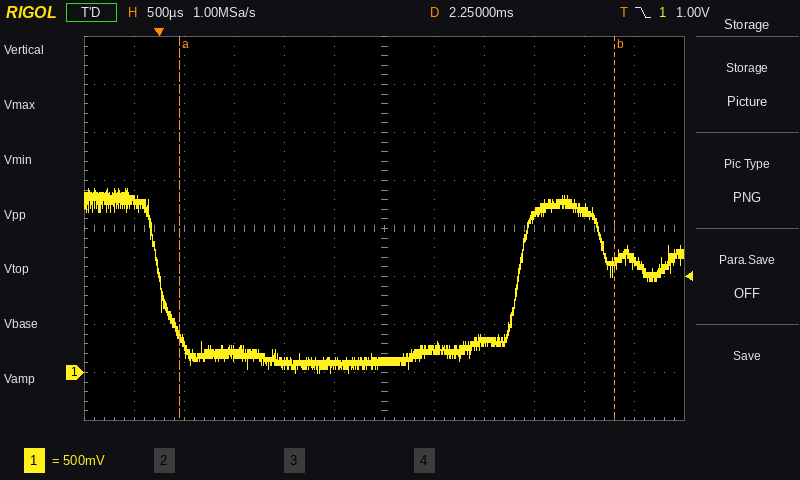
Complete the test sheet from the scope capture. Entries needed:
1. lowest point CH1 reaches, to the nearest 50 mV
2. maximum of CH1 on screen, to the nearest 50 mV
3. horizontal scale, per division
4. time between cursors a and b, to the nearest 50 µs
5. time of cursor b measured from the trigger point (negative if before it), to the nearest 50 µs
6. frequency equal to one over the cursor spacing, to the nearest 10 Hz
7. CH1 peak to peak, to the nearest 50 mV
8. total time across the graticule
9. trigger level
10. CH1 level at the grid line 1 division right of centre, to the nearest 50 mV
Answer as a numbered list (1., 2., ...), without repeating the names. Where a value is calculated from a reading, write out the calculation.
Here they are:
1. 0 mV
2. 1.90 V
3. 500 µs
4. 4.35 ms
5. +4.55 ms
6. 1 / 4.35 ms ≈ 230 Hz
7. 1.90 V − (0 mV) = 1.90 V
8. 6 ms
9. 1.00 V
10. 250 mV
